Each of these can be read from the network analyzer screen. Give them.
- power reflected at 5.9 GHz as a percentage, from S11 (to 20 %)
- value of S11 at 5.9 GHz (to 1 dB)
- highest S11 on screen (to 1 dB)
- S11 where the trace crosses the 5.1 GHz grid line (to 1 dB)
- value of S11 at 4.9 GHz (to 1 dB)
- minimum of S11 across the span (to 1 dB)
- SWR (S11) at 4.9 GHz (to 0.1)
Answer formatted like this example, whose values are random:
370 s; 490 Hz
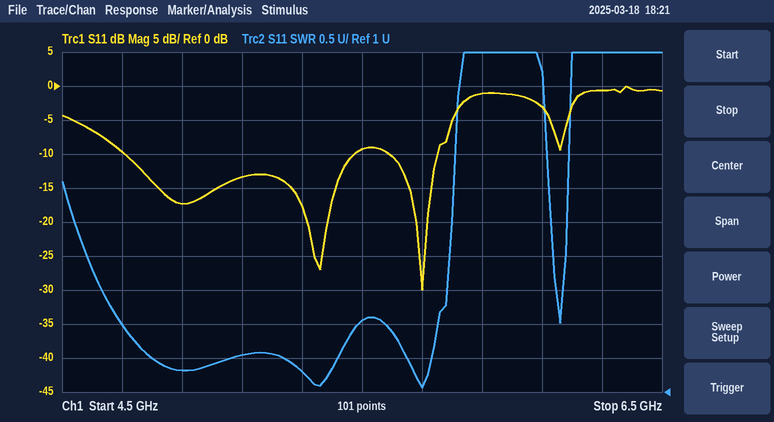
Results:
80 %; -1 dB; 0 dB; -13 dB; -17 dB; -30 dB; 1.3
